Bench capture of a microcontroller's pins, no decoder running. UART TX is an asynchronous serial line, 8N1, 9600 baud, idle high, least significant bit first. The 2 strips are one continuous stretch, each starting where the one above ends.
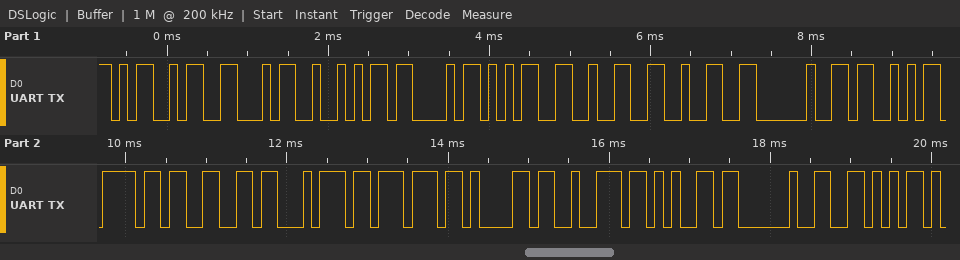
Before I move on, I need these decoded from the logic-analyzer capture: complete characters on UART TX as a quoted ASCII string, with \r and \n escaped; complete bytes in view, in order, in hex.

"MFRC522 Software V"
4D 46 52 43 35 32 32 20 53 6F 66 74 77 61 72 65 20 56
